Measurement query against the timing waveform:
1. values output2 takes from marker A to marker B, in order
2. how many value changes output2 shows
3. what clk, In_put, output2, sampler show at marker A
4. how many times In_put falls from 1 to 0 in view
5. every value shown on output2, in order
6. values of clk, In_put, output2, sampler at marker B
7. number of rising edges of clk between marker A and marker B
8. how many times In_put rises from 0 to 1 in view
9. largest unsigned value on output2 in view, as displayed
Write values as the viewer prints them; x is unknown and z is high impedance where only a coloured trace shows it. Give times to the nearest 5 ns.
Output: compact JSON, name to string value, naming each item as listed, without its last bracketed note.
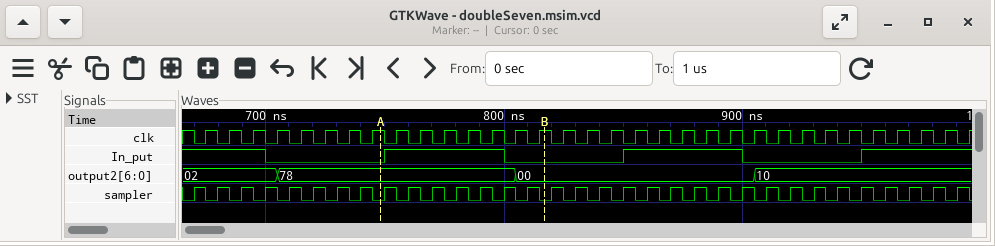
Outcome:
{"values output2 takes from marker A to marker B, in order": "78, 00", "how many value changes output2 shows": "3", "what clk, In_put, output2, sampler show at marker A": "clk=1, In_put=0, output2=78, sampler=0", "how many times In_put falls from 1 to 0 in view": "3", "every value shown on output2, in order": "02, 78, 00, 10", "values of clk, In_put, output2, sampler at marker B": "clk=1, In_put=0, output2=00, sampler=0", "number of rising edges of clk between marker A and marker B": "7", "how many times In_put rises from 0 to 1 in view": "3", "largest unsigned value on output2 in view, as displayed": "78"}
